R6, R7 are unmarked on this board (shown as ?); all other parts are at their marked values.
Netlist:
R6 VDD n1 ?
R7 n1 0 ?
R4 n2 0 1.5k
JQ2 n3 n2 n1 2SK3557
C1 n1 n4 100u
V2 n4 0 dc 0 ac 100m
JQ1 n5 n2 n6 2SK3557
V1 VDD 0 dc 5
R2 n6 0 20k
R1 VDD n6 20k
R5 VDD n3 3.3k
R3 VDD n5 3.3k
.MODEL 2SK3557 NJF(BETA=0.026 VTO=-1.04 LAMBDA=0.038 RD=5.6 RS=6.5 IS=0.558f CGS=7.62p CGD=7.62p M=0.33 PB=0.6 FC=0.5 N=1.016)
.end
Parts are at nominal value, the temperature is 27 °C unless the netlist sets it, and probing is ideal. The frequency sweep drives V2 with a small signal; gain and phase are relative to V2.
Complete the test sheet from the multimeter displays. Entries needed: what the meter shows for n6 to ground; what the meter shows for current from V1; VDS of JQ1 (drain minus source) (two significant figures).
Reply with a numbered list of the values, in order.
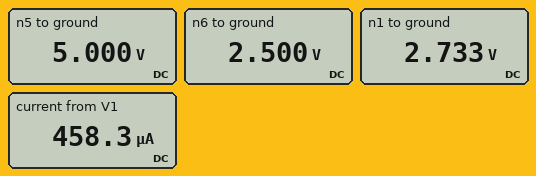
1. 2.500 V
2. 458.3 µA
3. 2.5 V
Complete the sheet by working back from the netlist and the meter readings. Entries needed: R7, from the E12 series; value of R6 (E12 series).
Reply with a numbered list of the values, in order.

1. 8.2 kΩ
2. 6.8 kΩ
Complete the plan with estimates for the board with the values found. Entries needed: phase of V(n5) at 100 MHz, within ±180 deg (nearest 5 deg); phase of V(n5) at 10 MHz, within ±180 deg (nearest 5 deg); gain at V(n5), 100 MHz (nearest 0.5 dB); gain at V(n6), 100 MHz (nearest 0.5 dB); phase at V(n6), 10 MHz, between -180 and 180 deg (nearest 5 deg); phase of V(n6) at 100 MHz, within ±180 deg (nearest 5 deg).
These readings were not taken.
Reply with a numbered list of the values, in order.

1. 45 deg
2. 125 deg
3. -2.0 dB
4. -2.0 dB
5. 85 deg
6. 35 deg
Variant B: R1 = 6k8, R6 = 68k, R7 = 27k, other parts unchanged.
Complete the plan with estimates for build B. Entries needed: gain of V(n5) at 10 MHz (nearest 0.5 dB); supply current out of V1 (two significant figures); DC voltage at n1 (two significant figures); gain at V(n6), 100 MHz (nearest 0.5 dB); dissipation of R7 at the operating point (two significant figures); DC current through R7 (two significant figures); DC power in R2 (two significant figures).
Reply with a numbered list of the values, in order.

1. -19.0 dB
2. 240 µA
3. 1.4 V
4. -1.5 dB
5. 75 µW
6. 53 µA
7. 700 µW
